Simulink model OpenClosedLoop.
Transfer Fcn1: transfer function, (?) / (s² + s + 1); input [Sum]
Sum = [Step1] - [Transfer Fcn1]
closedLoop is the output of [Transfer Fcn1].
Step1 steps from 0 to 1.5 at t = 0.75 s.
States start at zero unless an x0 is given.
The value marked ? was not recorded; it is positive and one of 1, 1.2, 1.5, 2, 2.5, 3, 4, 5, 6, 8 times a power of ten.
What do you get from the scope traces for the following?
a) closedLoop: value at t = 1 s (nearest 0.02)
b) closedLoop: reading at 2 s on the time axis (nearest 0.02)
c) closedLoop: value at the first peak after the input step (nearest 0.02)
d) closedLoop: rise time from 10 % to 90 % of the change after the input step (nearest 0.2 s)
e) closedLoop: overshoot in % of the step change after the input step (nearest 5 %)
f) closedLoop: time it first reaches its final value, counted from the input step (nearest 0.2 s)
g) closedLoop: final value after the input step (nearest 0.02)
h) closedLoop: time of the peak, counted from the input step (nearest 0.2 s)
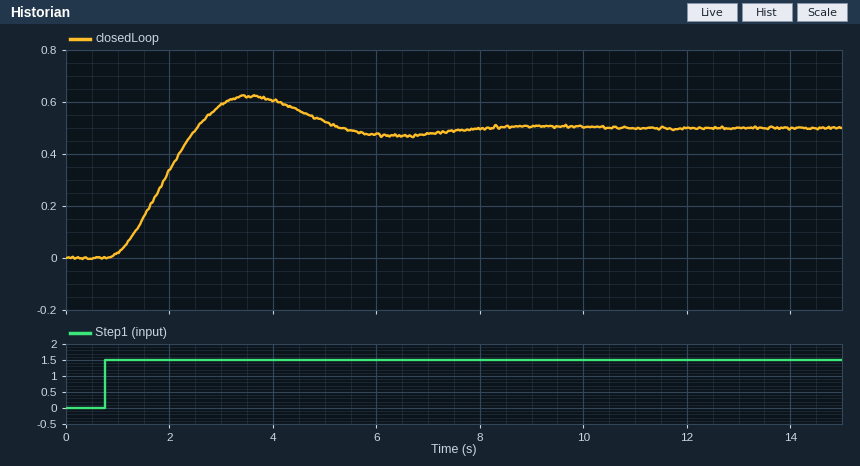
0.02
0.34
0.62
1.2 s
25 %
1.8 s
0.50
2.8 s
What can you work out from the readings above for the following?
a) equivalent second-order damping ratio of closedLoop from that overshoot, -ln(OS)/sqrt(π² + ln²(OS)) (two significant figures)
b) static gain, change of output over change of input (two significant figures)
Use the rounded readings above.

0.40
0.33
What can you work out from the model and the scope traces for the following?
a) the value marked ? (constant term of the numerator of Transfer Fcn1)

0.5
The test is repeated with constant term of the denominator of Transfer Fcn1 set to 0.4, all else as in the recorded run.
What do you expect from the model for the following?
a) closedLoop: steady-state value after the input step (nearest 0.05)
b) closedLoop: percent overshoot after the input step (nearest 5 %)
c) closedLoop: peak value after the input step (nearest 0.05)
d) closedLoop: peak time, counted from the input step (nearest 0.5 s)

0.85
15 %
0.95
4.0 s
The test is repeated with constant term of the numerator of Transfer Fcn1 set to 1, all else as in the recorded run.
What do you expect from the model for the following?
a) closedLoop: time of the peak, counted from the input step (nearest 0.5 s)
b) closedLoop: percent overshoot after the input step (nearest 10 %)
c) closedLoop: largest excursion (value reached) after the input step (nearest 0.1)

2.5 s
30 %
1.0
